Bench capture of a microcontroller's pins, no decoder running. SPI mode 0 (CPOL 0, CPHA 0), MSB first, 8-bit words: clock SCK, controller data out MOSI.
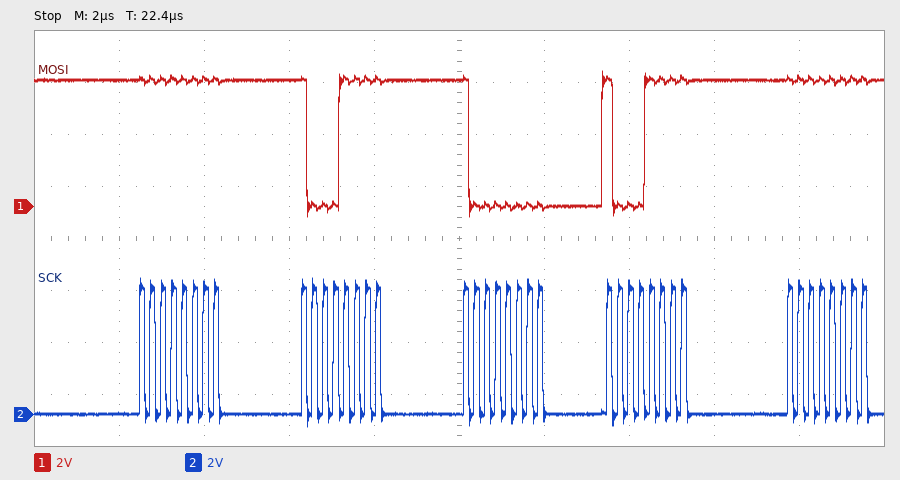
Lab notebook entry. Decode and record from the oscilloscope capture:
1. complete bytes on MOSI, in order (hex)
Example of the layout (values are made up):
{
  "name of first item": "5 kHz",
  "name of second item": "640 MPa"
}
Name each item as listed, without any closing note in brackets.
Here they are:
{
  "complete bytes on MOSI, in order": "0xFF 0x8F 0x80 0x8F 0xFF"
}
